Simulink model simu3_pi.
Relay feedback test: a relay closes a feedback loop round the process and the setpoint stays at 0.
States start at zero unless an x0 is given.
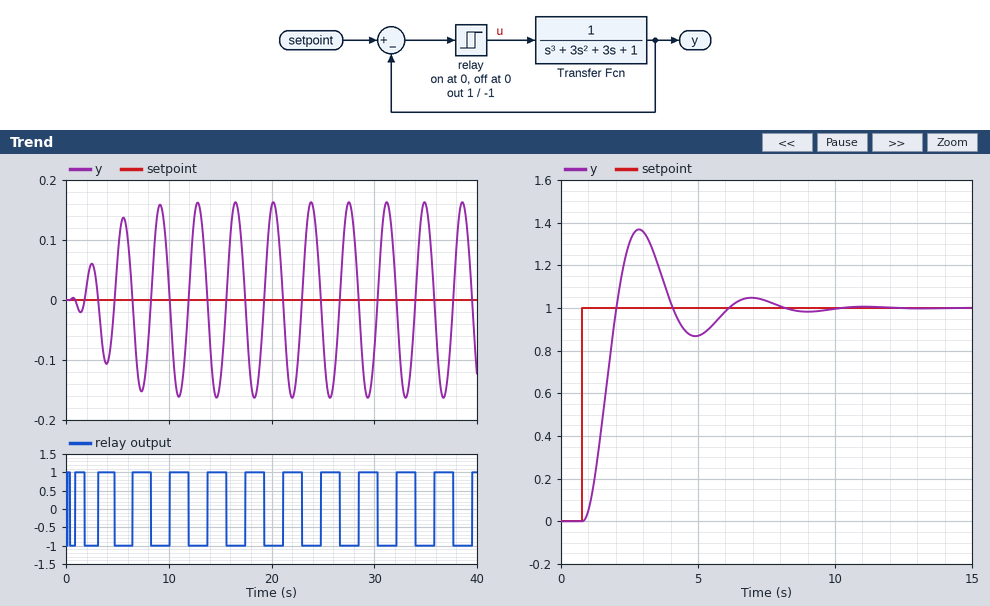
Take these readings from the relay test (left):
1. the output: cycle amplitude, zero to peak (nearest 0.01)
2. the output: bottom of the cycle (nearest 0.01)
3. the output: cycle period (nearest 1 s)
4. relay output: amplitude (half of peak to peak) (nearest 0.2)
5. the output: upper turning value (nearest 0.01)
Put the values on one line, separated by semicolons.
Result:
0.16; -0.16; 4 s; 1.0; 0.16
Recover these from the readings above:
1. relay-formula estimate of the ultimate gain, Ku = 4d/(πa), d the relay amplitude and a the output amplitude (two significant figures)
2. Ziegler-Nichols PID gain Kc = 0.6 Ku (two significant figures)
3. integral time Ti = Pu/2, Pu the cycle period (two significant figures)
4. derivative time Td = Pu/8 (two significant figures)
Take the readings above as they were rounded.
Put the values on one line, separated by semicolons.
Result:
8.0; 4.8; 2.0 s; 0.50 s
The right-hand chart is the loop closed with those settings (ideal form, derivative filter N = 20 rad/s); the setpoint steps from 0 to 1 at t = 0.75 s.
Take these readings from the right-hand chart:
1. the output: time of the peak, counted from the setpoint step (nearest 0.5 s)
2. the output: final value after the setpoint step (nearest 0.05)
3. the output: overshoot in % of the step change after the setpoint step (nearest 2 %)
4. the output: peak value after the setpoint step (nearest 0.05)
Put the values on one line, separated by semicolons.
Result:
2.0 s; 1.00; 36 %; 1.35
